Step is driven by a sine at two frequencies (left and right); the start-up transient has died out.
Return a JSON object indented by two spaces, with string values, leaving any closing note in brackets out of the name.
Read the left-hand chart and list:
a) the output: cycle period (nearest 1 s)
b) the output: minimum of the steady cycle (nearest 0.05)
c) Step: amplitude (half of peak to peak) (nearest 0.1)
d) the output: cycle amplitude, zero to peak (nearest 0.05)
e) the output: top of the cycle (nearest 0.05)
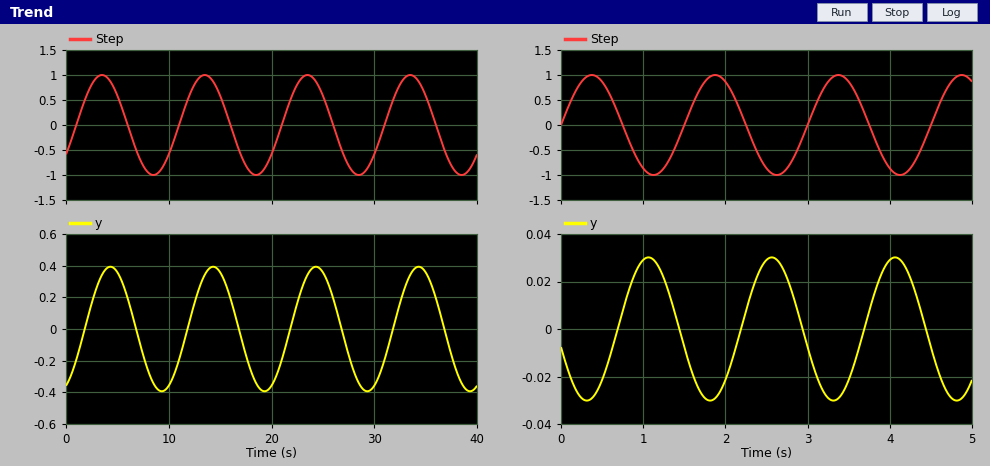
{
  "the output: cycle period": "10 s",
  "the output: minimum of the steady cycle": "-0.40",
  "Step: amplitude (half of peak to peak)": "1.0",
  "the output: cycle amplitude, zero to peak": "0.40",
  "the output: top of the cycle": "0.40"
}
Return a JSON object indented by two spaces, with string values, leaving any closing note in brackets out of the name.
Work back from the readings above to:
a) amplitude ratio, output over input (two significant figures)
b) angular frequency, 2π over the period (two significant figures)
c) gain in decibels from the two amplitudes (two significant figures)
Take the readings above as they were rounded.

{
  "amplitude ratio, output over input": "0.40",
  "angular frequency, 2π over the period": "0.63 rad/s",
  "gain in decibels from the two amplitudes": "-8.0 dB"
}
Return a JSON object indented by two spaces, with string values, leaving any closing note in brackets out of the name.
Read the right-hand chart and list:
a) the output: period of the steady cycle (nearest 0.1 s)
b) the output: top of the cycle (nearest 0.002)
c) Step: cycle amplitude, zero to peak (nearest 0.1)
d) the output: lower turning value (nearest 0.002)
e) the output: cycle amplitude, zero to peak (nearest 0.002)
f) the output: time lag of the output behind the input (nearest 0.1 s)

{
  "the output: period of the steady cycle": "1.5 s",
  "the output: top of the cycle": "0.030",
  "Step: cycle amplitude, zero to peak": "1.0",
  "the output: lower turning value": "-0.030",
  "the output: cycle amplitude, zero to peak": "0.030",
  "the output: time lag of the output behind the input": "0.7 s"
}
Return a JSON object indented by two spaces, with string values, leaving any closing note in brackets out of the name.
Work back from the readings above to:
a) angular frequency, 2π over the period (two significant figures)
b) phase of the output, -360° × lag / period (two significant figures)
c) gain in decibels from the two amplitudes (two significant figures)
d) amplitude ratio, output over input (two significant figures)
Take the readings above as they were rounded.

{
  "angular frequency, 2π over the period": "4.2 rad/s",
  "phase of the output, -360° × lag / period": "-170°",
  "gain in decibels from the two amplitudes": "-30 dB",
  "amplitude ratio, output over input": "0.030"
}
